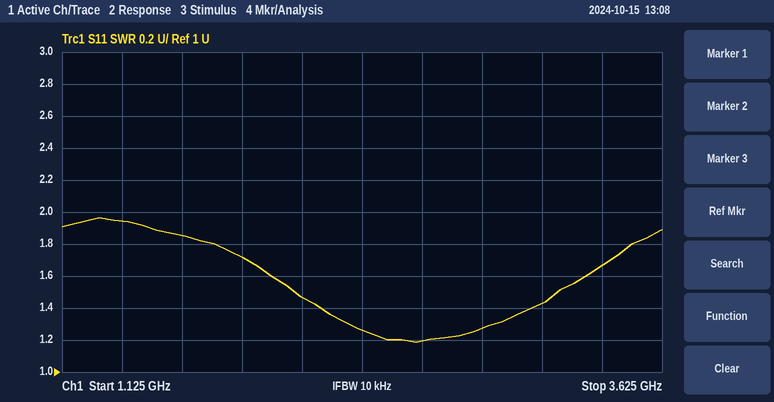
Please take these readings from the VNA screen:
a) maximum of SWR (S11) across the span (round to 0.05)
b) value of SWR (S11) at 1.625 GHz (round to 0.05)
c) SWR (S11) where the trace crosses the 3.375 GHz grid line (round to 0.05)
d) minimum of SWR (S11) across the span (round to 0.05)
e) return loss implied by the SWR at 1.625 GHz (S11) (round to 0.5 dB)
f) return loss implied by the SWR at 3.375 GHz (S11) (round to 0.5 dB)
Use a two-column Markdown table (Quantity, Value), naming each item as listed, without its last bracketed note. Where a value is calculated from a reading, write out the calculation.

| Quantity | Value |
|---|---|
| maximum of SWR (S11) across the span | 1.95 |
| value of SWR (S11) at 1.625 GHz | 1.85 |
| SWR (S11) where the trace crosses the 3.375 GHz grid line | 1.65 |
| minimum of SWR (S11) across the span | 1.20 |
| return loss implied by the SWR at 1.625 GHz (S11) | −20 log10((1.85 − 1)/(1.85 + 1)) ≈ 10.5 dB |
| return loss implied by the SWR at 3.375 GHz (S11) | −20 log10((1.65 − 1)/(1.65 + 1)) ≈ 12.2 dB, so 12.0 dB to the nearest 0.5 dB |
